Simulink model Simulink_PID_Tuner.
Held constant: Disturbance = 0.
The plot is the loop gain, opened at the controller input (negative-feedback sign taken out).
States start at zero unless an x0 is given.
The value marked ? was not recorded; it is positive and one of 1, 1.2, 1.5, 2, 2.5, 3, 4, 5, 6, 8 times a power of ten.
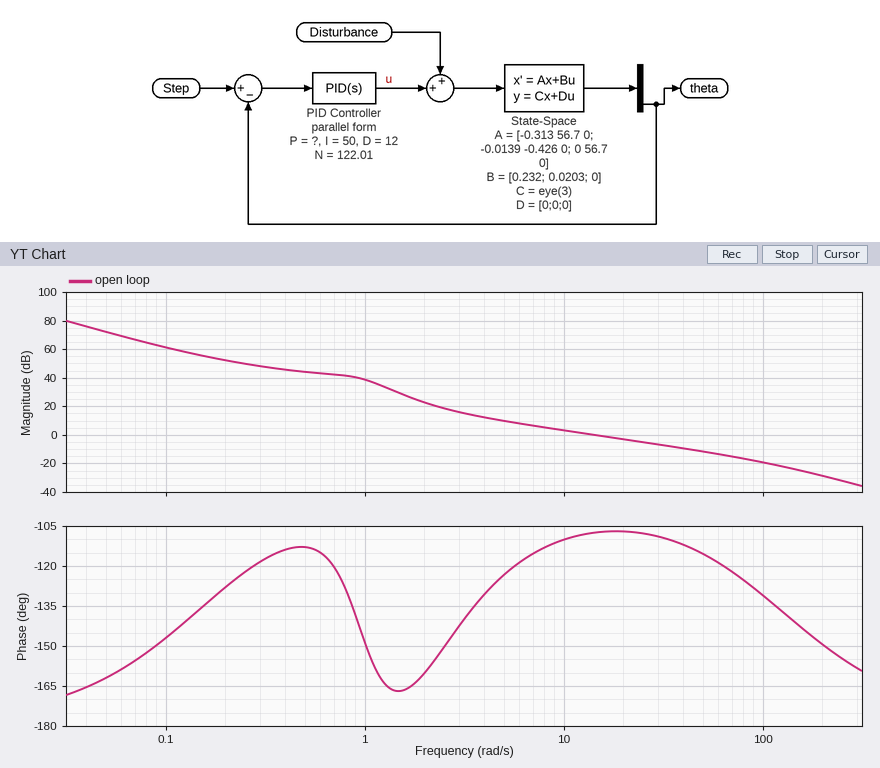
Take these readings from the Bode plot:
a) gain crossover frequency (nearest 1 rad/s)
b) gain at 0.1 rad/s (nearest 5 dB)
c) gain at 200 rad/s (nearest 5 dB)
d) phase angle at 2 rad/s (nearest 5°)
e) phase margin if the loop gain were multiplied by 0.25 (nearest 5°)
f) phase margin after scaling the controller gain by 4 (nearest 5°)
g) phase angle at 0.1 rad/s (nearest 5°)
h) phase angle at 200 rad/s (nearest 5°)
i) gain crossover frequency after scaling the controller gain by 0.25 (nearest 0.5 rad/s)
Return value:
14 rad/s
60 dB
-30 dB
-160°
50°
65°
-145°
-150°
4.0 rad/s
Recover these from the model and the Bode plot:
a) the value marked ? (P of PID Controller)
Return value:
40
